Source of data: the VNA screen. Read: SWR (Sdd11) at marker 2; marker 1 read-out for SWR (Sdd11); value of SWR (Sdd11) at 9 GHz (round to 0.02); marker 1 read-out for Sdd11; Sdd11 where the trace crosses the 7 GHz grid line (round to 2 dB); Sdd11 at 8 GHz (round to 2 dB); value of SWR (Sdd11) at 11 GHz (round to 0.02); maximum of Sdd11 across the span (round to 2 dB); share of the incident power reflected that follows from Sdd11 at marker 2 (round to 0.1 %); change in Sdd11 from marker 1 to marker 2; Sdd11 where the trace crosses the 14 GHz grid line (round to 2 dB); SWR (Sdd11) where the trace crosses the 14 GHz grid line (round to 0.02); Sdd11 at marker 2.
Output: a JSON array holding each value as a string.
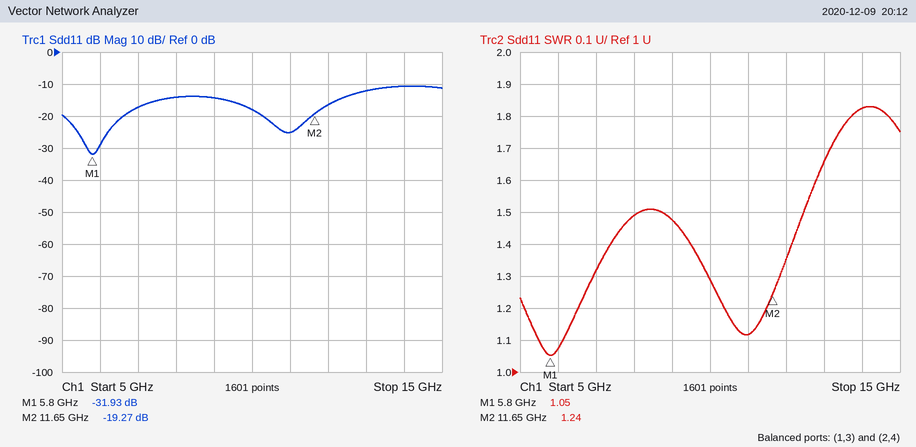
["1.24", "1.05", "1.48", "-31.93 dB", "-18 dB", "-14 dB", "1.12", "-10 dB", "1.2 %", "12.66 dB", "-10 dB", "1.82", "-19.27 dB"]
